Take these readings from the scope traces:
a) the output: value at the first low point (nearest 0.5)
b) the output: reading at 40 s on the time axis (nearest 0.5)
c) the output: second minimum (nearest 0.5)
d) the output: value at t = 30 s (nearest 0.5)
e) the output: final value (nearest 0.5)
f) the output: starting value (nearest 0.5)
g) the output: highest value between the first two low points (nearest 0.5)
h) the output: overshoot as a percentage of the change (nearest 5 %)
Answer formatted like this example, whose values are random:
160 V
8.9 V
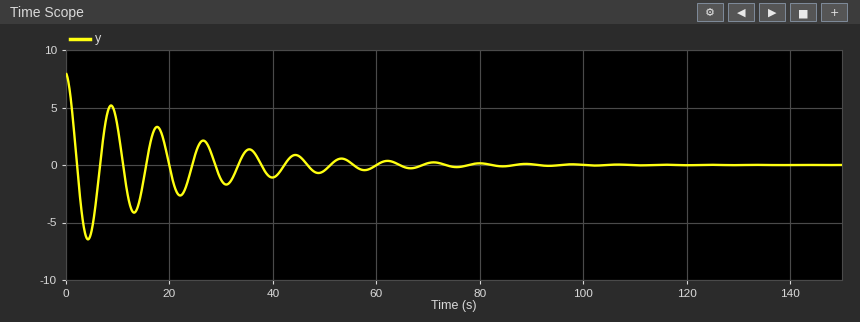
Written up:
-6.5
-1.0
-4.0
-1.5
0.0
8.0
5.0
80 %
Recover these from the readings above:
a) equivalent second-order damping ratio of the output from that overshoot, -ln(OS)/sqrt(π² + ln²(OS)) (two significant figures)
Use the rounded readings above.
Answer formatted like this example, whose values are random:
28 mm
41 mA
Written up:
0.071
